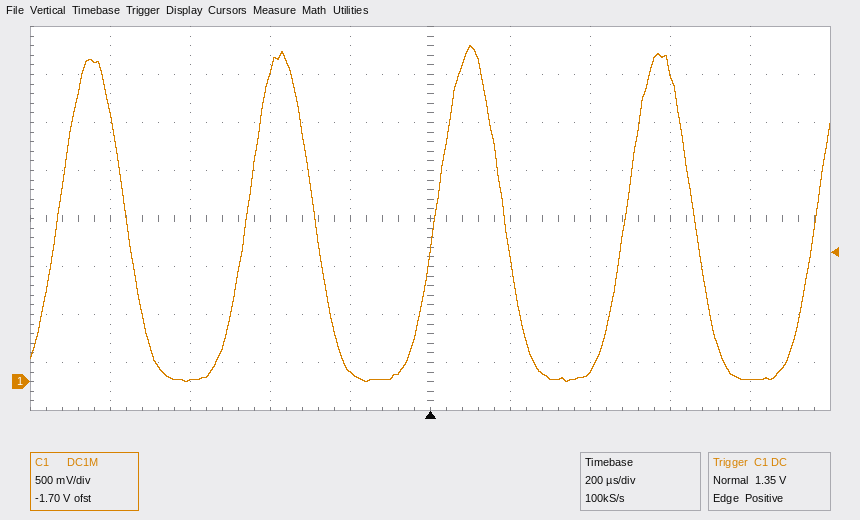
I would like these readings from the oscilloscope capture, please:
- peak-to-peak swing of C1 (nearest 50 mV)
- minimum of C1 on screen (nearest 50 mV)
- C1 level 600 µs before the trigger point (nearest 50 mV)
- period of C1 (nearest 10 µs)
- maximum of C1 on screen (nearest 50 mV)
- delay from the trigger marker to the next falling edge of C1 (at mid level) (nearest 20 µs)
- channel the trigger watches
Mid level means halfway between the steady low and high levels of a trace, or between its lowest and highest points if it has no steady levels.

3.50 V
0 mV
0 mV
470 µs
3.50 V
180 µs
C1
